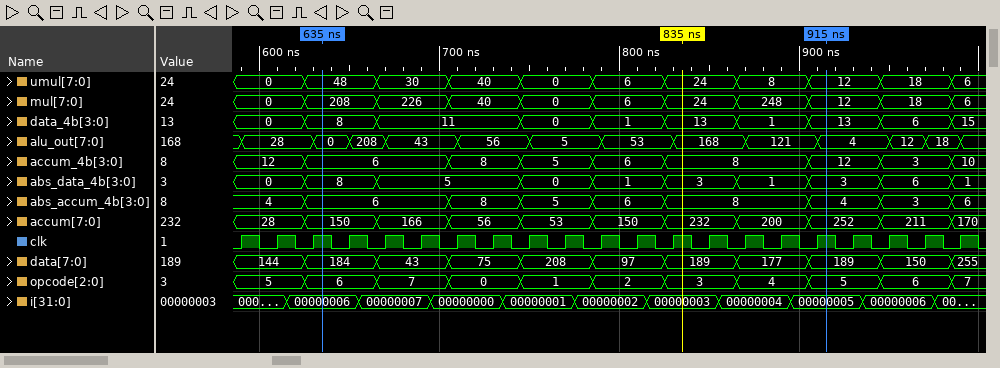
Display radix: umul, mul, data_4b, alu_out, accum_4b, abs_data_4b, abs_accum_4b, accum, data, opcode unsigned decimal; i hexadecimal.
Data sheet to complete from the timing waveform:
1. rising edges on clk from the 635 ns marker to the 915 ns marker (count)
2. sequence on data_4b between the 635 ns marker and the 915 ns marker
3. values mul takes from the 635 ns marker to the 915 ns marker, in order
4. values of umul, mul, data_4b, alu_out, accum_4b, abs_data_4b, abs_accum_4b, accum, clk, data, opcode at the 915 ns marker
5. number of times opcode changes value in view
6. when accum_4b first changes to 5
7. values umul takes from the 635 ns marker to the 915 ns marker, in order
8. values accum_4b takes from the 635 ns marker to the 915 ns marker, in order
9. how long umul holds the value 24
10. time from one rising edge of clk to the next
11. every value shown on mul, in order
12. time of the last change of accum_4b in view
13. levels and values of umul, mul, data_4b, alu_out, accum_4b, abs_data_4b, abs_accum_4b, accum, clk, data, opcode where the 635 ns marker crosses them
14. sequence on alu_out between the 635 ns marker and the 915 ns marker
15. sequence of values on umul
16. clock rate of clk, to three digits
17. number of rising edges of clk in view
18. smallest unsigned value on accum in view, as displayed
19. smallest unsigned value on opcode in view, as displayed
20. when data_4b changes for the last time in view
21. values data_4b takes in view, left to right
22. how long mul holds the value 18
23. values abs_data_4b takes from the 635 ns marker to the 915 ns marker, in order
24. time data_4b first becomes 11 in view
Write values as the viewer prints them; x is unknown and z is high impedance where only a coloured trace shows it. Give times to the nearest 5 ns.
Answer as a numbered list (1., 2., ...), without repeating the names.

1. 14
2. 8, 11, 0, 1, 13, 1, 13
3. 208, 226, 40, 0, 6, 24, 248, 12
4. umul=12, mul=12, data_4b=13, alu_out=4, accum_4b=12, abs_data_4b=3, abs_accum_4b=4, accum=252, clk=1, data=189, opcode=5
5. 10
6. 745 ns
7. 48, 30, 40, 0, 6, 24, 8, 12
8. 6, 8, 5, 6, 8, 12
9. 40 ns
10. 20 ns
11. 0, 208, 226, 40, 0, 6, 24, 248, 12, 18, 6
12. 985 ns
13. umul=48, mul=208, data_4b=8, alu_out=0, accum_4b=6, abs_data_4b=8, abs_accum_4b=6, accum=150, clk=1, data=184, opcode=6
14. 0, 208, 43, 56, 5, 53, 168, 121, 4
15. 0, 48, 30, 40, 0, 6, 24, 8, 12, 18, 6
16. 50.0 MHz
17. 21
18. 28
19. 0
20. 985 ns
21. 0, 8, 11, 0, 1, 13, 1, 13, 6, 15
22. 40 ns
23. 8, 5, 0, 1, 3, 1, 3
24. 665 ns
